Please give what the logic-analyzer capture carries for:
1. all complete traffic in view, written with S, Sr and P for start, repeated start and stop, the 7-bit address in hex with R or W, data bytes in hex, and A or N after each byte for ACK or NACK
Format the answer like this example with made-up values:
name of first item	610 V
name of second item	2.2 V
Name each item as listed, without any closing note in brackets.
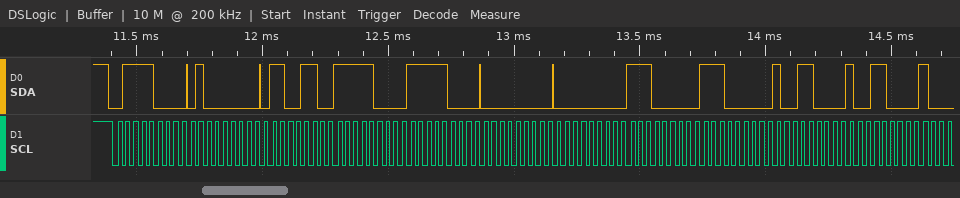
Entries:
all complete traffic in view, written with S, Sr and P for start, repeated start and stop, the 7-bit address in hex with R or W, data bytes in hex, and A or N after each byte for ACK or NACK	S 3CW A 40 A 66 A F8 A F8 A 00 A 00 A E0 A E0 A 98 A 98 A
